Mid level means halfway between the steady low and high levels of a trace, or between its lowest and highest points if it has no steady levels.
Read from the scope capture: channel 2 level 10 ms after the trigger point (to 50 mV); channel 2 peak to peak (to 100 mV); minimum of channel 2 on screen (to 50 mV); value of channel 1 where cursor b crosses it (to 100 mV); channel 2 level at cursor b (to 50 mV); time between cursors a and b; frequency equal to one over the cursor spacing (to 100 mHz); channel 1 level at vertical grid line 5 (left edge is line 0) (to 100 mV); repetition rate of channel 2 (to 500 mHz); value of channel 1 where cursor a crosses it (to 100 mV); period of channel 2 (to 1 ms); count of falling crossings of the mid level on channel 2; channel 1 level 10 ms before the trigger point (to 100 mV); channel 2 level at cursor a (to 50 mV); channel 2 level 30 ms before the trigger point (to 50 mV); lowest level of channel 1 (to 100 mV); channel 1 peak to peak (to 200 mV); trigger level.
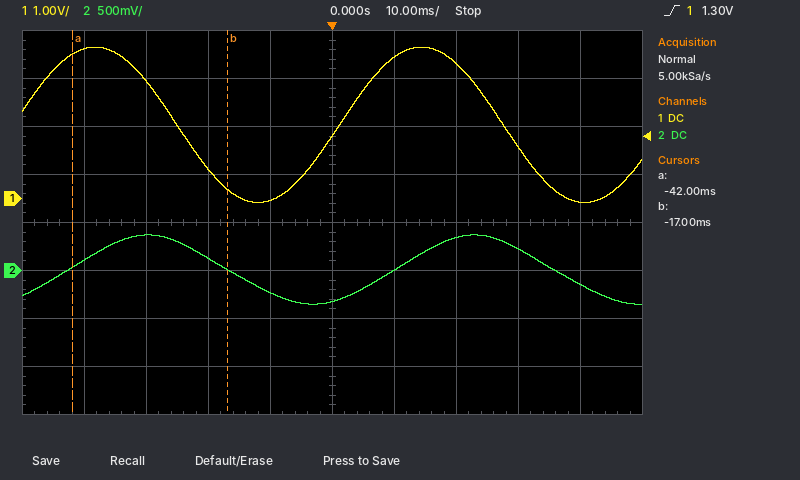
0 mV
700 mV
-350 mV
200 mV
0 mV
25 ms
40.0 Hz
1.3 V
19.0 Hz
3.0 V
53 ms
2
0.0 V
50 mV
350 mV
-100 mV
3.2 V
1.30 V
